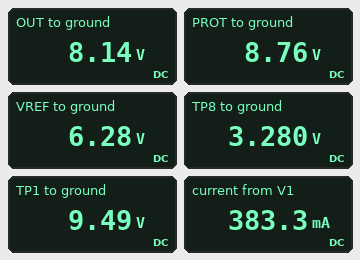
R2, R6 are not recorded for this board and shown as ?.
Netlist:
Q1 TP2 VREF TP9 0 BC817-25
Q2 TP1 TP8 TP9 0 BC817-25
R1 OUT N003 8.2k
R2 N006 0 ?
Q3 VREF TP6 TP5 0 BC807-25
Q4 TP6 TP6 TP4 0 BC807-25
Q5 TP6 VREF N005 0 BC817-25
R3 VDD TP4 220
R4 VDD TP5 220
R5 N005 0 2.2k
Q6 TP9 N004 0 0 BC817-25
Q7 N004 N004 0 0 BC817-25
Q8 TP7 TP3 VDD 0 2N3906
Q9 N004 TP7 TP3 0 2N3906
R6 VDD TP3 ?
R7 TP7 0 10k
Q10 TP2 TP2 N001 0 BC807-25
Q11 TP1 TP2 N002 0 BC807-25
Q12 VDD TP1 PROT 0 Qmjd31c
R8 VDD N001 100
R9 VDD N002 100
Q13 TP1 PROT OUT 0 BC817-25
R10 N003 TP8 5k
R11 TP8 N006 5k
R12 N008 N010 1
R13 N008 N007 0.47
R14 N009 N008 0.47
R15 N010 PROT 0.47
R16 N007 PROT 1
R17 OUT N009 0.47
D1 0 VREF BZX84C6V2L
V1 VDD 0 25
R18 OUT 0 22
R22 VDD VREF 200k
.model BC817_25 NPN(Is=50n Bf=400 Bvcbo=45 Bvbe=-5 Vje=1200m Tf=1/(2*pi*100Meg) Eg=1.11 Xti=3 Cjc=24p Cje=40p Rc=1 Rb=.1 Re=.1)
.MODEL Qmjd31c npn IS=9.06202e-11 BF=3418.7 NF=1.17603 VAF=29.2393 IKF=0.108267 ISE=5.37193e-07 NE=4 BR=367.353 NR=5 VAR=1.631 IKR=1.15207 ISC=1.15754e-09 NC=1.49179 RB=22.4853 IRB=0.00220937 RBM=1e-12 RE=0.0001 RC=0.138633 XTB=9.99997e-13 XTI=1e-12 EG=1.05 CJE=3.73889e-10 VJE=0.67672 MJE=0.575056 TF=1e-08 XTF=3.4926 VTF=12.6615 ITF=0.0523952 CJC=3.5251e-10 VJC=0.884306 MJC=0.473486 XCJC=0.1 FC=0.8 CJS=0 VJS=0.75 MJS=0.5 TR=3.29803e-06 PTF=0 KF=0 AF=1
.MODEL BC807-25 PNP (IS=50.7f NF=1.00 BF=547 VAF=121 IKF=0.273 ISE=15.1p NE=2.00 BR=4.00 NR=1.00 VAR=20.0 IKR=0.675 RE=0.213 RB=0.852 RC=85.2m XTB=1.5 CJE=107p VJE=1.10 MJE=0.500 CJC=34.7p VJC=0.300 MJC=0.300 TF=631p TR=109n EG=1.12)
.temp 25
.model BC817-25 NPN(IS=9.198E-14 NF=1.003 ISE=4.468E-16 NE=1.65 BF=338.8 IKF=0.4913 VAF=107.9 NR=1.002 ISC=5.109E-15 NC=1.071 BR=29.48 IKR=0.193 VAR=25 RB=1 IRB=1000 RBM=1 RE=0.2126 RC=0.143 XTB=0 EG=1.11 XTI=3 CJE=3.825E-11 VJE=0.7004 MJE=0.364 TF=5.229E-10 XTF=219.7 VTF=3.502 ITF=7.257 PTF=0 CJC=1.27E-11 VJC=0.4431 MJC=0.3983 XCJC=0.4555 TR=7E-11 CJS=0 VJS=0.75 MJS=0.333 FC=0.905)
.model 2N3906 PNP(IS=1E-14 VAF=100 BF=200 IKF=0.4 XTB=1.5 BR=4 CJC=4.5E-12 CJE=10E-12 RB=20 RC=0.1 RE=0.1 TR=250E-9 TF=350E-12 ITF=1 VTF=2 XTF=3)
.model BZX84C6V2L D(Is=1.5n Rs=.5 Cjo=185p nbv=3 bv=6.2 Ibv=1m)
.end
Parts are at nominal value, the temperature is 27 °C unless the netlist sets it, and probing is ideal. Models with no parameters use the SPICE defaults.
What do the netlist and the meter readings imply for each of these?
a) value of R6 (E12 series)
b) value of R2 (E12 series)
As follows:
270 Ω
3.9 kΩ
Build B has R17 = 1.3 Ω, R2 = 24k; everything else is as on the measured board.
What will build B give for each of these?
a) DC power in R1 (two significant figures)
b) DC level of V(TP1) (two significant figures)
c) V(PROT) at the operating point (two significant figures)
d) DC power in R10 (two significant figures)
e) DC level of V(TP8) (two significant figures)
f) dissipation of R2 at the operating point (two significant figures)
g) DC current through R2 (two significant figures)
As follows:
140 µW
6.8 V
6.1 V
85 µW
3.8 V
410 µW
130 µA
